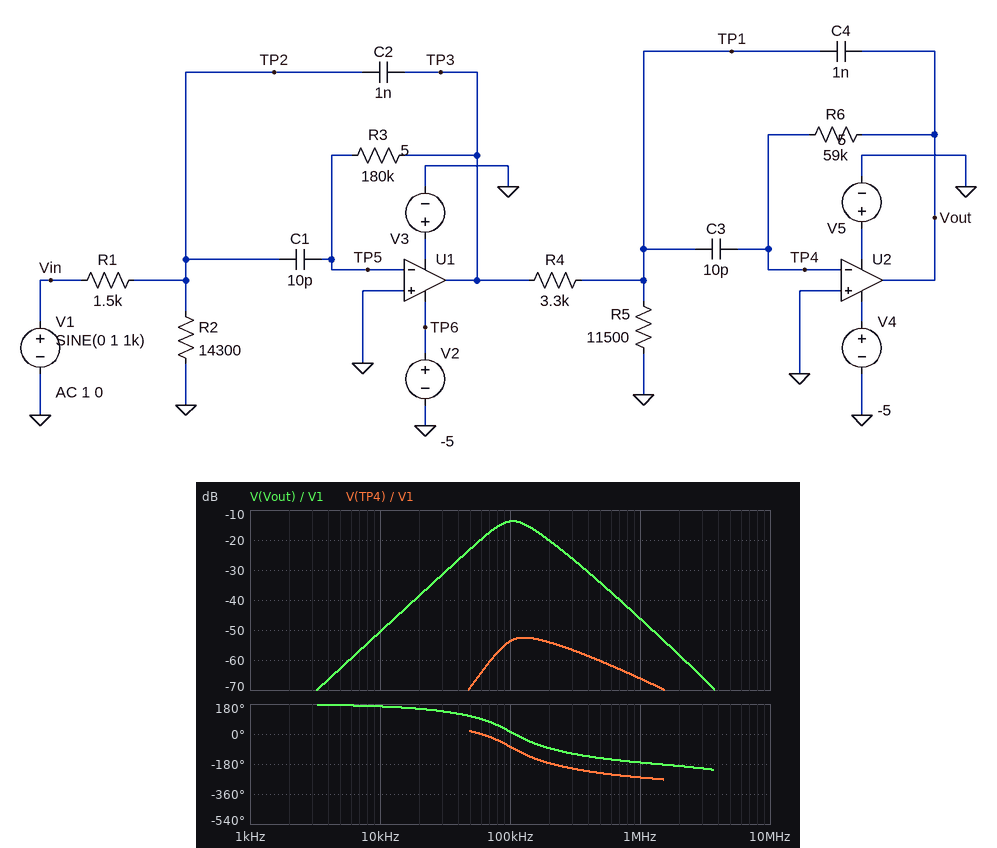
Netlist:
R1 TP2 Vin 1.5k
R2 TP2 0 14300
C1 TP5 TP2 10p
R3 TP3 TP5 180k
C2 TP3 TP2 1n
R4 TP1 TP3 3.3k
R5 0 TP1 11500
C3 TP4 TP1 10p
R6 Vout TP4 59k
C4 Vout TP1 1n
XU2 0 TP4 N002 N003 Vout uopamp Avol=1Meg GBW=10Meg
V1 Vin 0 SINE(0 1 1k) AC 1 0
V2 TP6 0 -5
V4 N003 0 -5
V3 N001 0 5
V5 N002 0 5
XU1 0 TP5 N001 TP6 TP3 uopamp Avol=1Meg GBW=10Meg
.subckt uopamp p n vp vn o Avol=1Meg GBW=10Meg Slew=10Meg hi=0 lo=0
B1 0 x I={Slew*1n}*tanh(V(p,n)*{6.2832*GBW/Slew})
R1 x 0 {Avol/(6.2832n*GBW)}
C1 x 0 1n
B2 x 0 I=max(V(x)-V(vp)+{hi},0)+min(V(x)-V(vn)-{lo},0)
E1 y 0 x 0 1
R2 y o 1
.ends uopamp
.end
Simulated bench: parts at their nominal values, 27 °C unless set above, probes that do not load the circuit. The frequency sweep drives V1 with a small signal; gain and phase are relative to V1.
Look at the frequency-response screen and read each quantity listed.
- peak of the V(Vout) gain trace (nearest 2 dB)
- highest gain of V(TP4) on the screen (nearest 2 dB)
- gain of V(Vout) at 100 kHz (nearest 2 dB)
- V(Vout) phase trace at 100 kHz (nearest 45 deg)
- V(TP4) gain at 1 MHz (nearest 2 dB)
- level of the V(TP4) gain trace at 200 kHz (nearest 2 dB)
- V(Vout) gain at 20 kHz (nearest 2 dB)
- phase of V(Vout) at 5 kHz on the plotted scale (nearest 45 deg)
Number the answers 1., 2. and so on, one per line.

1. -14 dB
2. -52 dB
3. -14 dB
4. 0 deg
5. -66 dB
6. -54 dB
7. -38 dB
8. 180 deg
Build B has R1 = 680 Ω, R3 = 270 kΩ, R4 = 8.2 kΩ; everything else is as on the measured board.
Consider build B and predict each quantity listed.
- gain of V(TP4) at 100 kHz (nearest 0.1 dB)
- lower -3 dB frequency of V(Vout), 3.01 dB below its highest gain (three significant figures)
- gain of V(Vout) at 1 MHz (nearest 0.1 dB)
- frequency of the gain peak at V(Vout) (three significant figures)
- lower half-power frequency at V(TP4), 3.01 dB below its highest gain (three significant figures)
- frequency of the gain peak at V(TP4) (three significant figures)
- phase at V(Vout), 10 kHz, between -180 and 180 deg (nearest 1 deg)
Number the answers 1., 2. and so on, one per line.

1. -52.8 dB
2. 92.7 kHz
3. -47.3 dB
4. 118 kHz
5. 101 kHz
6. 125 kHz
7. 160 deg
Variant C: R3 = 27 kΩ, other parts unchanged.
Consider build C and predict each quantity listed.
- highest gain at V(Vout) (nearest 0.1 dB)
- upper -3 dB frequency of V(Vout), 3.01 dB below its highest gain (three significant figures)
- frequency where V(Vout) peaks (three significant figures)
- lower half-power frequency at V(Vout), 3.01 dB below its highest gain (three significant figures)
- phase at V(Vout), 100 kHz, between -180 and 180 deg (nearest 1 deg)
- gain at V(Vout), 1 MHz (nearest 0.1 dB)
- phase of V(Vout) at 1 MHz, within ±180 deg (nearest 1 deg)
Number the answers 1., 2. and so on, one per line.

1. -30.9 dB
2. 354 kHz
3. 179 kHz
4. 91.9 kHz
5. 57 deg
6. -47.1 dB
7. -144 deg
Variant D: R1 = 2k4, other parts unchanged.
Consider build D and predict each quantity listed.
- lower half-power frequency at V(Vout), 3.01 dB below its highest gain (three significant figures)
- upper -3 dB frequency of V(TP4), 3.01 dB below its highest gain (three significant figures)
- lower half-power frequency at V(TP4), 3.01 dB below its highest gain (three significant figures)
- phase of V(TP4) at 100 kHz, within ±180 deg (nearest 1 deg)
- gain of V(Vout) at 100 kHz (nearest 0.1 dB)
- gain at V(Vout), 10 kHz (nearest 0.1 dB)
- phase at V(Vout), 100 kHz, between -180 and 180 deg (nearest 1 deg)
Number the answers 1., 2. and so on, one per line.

1. 59.4 kHz
2. 291 kHz
3. 77.8 kHz
4. -97 deg
5. -18.4 dB
6. -51.1 dB
7. -7 deg
